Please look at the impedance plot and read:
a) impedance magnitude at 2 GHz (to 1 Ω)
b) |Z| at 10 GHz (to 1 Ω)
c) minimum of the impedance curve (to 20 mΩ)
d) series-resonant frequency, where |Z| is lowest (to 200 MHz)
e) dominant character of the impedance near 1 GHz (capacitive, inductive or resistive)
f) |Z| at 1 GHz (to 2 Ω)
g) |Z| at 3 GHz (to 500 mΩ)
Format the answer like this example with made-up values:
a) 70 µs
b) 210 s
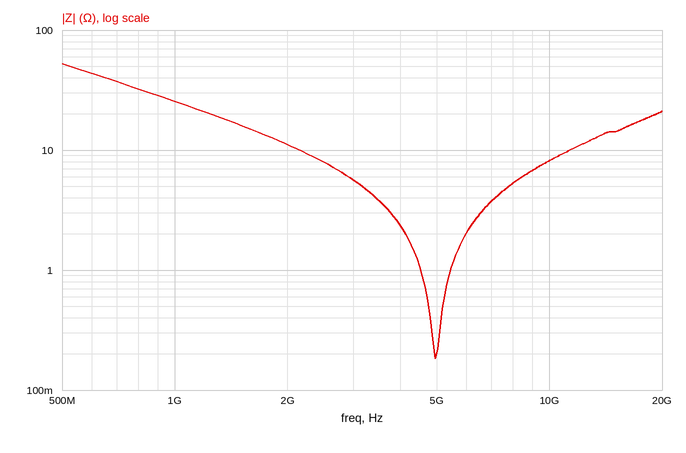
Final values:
a) 11 Ω
b) 8 Ω
c) 180 mΩ
d) 5.0 GHz
e) capacitive
f) 26 Ω
g) 5.5 Ω
